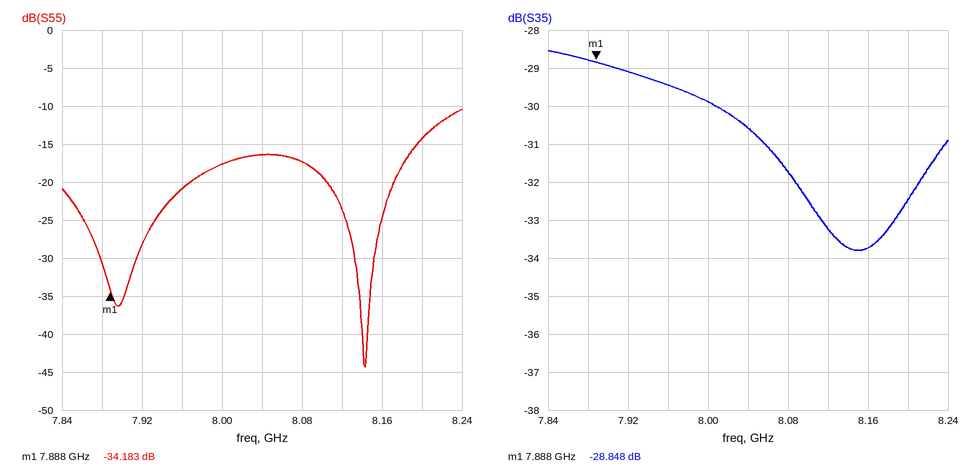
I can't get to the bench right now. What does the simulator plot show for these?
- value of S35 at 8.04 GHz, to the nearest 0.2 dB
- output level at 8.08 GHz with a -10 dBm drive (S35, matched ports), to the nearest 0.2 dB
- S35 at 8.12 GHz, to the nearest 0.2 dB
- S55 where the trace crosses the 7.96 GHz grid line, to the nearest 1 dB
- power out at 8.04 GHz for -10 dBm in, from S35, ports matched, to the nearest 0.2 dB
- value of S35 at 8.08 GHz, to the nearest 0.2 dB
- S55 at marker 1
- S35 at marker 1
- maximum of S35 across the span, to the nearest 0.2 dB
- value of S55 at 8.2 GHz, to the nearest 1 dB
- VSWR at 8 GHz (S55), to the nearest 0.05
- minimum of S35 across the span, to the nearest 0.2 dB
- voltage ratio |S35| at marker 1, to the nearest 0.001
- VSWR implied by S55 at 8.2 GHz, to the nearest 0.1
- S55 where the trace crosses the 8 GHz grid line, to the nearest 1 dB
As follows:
-30.6 dB
-41.8 dBm
-33.2 dB
-21 dB
-40.6 dBm
-31.8 dB
-34.183 dB
-28.848 dB
-28.6 dB
-14 dB
1.30
-33.8 dB
0.036
1.5
-18 dB
